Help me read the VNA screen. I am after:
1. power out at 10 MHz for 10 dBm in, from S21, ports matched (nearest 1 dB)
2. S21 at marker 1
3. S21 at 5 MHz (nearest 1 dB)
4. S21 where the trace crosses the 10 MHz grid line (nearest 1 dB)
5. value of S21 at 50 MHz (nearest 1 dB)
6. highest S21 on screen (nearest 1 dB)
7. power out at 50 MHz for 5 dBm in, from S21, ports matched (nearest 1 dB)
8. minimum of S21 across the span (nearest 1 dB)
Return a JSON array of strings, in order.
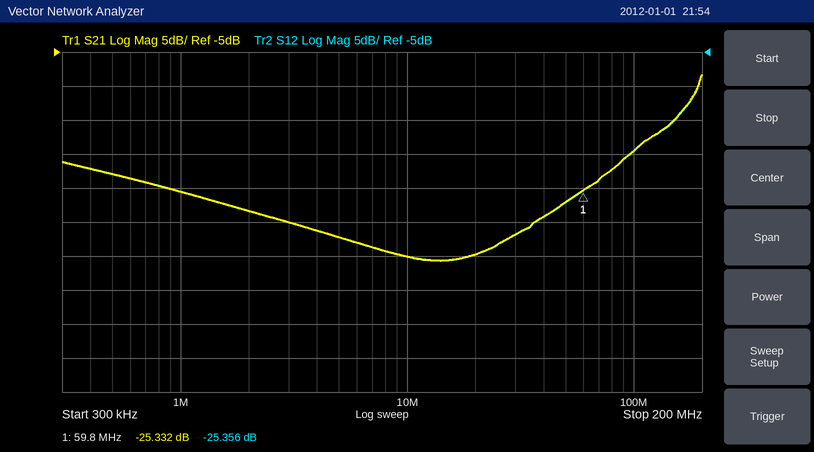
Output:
["-25 dBm", "-25.332 dB", "-32 dB", "-35 dB", "-27 dB", "-8 dB", "-22 dBm", "-36 dB"]
